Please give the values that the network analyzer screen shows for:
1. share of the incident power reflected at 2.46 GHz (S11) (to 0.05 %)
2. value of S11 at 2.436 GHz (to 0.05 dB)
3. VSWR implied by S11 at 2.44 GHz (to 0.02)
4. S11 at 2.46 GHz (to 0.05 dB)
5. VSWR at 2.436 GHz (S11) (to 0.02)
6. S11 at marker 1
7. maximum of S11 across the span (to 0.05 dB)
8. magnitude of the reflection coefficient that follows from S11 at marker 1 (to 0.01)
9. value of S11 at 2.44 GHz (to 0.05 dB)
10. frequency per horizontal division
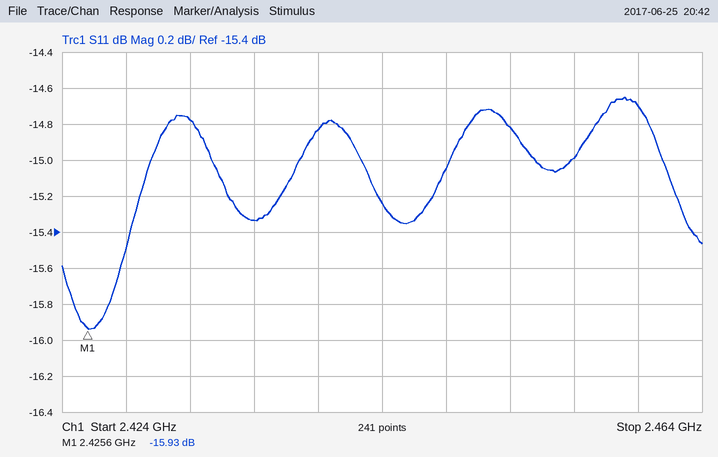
3.40 %
-15.35 dB
1.44
-14.70 dB
1.42
-15.93 dB
-14.65 dB
0.16
-14.85 dB
4 MHz
